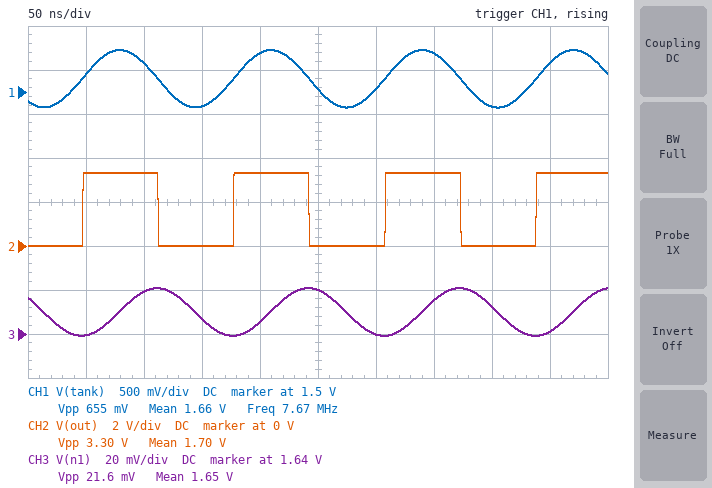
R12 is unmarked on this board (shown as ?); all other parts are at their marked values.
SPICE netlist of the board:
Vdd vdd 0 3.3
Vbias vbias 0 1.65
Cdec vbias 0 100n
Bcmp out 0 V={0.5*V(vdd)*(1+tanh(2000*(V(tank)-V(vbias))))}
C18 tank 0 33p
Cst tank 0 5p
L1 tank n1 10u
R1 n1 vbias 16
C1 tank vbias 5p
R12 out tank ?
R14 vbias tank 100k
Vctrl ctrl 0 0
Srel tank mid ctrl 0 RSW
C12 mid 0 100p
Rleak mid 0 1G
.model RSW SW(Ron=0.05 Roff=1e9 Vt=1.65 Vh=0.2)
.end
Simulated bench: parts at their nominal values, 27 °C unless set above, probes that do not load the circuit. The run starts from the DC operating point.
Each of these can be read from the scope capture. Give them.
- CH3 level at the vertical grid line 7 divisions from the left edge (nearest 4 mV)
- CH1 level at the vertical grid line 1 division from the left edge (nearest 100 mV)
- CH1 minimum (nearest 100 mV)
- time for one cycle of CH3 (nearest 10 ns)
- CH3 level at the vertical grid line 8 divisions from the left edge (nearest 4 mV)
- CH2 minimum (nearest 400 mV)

1.656 V
1.7 V
1.3 V
130 ns
1.652 V
0 V
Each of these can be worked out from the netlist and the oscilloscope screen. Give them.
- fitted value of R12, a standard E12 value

68 kΩ
